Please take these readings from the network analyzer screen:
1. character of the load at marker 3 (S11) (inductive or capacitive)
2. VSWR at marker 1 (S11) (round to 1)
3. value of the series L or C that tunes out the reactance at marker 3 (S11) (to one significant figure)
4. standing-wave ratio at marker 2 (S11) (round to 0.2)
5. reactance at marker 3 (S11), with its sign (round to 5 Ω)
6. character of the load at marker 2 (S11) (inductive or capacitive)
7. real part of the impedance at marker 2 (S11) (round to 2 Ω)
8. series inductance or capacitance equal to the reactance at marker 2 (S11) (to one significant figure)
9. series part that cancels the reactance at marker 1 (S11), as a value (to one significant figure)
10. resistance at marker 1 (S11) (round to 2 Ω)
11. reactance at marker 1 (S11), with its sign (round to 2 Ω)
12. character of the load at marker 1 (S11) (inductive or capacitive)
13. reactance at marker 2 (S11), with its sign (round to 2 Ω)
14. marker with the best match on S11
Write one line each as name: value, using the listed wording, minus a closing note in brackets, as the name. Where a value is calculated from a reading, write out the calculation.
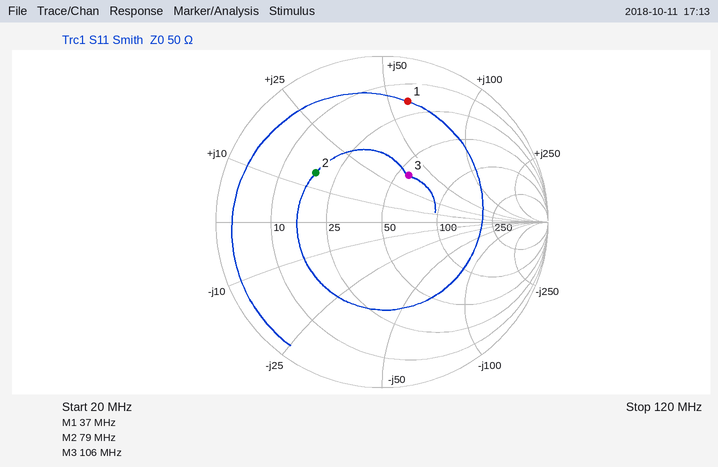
character of the load at marker 3 (S11): inductive
VSWR at marker 1 (S11): 7
value of the series L or C that tunes out the reactance at marker 3 (S11): C = 1/(2π × 106 MHz × 35 Ω) ≈ 42.9 pF, so 40 pF to one significant figure
standing-wave ratio at marker 2 (S11): 3.0
reactance at marker 3 (S11), with its sign: +35 Ω
character of the load at marker 2 (S11): inductive
real part of the impedance at marker 2 (S11): 18 Ω
series inductance or capacitance equal to the reactance at marker 2 (S11): L = 14 Ω/(2π × 79 MHz) ≈ 28.2 nH, so 30 nH to one significant figure
series part that cancels the reactance at marker 1 (S11), as a value: C = 1/(2π × 37 MHz × 58 Ω) ≈ 74.2 pF, so 70 pF to one significant figure
resistance at marker 1 (S11): 18 Ω
reactance at marker 1 (S11), with its sign: +58 Ω
character of the load at marker 1 (S11): inductive
reactance at marker 2 (S11), with its sign: +14 Ω
marker with the best match on S11: marker 3
